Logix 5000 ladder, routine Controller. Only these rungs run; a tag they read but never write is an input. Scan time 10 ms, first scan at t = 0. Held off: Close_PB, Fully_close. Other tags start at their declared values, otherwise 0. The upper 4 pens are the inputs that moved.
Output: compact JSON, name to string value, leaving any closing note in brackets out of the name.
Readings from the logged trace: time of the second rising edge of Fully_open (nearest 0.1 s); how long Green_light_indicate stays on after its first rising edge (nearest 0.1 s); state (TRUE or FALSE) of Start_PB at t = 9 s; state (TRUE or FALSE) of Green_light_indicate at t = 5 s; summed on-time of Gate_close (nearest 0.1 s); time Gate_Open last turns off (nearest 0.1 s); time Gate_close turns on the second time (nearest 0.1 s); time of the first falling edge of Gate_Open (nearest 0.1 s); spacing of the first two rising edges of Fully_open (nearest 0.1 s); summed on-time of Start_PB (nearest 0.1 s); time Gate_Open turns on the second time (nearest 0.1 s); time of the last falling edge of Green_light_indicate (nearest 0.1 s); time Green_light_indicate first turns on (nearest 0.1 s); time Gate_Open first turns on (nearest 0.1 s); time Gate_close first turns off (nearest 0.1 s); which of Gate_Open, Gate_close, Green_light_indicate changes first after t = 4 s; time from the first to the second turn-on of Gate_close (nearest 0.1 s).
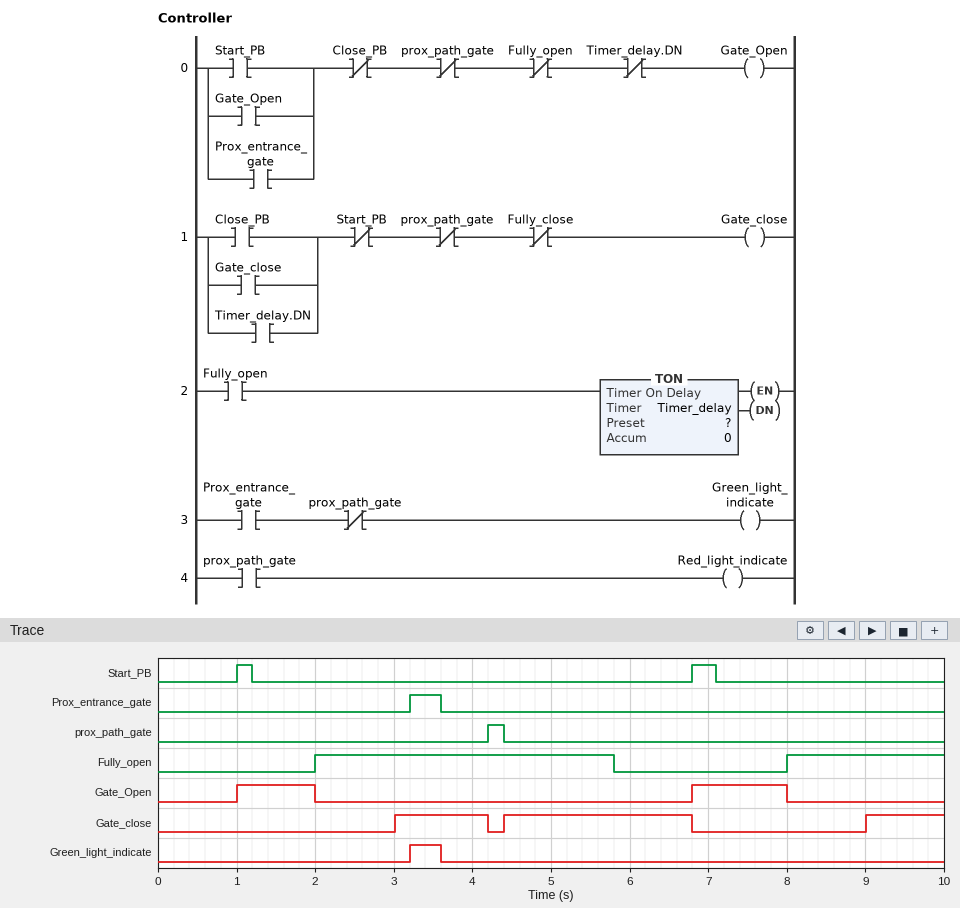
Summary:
{"time of the second rising edge of Fully_open": "8.0 s", "how long Green_light_indicate stays on after its first rising edge": "0.4 s", "state (TRUE or FALSE) of Start_PB at t = 9 s": "FALSE", "state (TRUE or FALSE) of Green_light_indicate at t = 5 s": "FALSE", "summed on-time of Gate_close": "4.6 s", "time Gate_Open last turns off": "8.0 s", "time Gate_close turns on the second time": "4.4 s", "time of the first falling edge of Gate_Open": "2.0 s", "spacing of the first two rising edges of Fully_open": "6.0 s", "summed on-time of Start_PB": "0.5 s", "time Gate_Open turns on the second time": "6.8 s", "time of the last falling edge of Green_light_indicate": "3.6 s", "time Green_light_indicate first turns on": "3.2 s", "time Gate_Open first turns on": "1.0 s", "time Gate_close first turns off": "4.2 s", "which of Gate_Open, Gate_close, Green_light_indicate changes first after t = 4 s": "Gate_close", "time from the first to the second turn-on of Gate_close": "1.4 s"}
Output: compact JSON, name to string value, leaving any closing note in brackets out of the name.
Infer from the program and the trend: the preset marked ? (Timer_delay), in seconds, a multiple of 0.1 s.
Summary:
{"the preset marked ? (Timer_delay), in seconds, a multiple of 0.1 s": "1.0 s"}
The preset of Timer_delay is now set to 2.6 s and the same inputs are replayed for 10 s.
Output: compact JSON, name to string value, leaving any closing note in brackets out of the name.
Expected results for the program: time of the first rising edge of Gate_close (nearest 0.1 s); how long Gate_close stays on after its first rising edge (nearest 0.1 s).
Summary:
{"time of the first rising edge of Gate_close": "4.6 s", "how long Gate_close stays on after its first rising edge": "2.2 s"}
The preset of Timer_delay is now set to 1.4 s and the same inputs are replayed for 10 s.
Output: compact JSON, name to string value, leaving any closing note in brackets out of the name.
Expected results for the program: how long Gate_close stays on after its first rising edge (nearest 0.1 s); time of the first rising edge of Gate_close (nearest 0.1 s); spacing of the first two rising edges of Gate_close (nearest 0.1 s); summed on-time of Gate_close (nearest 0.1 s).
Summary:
{"how long Gate_close stays on after its first rising edge": "0.8 s", "time of the first rising edge of Gate_close": "3.4 s", "spacing of the first two rising edges of Gate_close": "1.0 s", "summed on-time of Gate_close": "3.8 s"}
